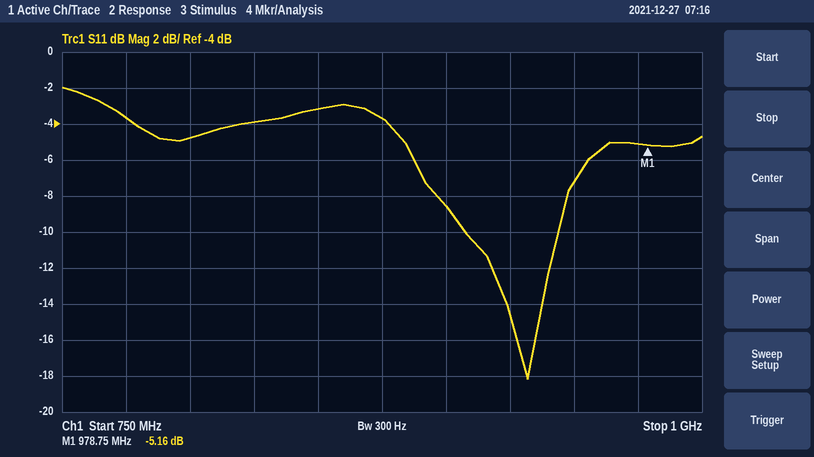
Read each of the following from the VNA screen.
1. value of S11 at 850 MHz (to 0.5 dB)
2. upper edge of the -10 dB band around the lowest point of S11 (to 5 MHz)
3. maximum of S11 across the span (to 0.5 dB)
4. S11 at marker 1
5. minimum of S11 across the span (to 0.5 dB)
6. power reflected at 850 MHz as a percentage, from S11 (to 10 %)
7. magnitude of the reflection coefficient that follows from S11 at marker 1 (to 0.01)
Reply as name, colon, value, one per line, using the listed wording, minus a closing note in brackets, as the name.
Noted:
value of S11 at 850 MHz: -3.0 dB
upper edge of the -10 dB band around the lowest point of S11: 945 MHz
maximum of S11 across the span: -2.0 dB
S11 at marker 1: -5.16 dB
minimum of S11 across the span: -18.0 dB
power reflected at 850 MHz as a percentage, from S11: 50 %
magnitude of the reflection coefficient that follows from S11 at marker 1: 0.55
